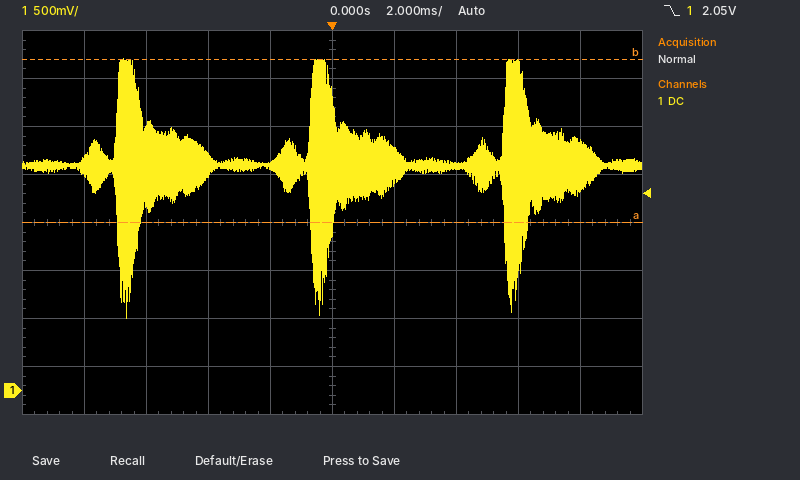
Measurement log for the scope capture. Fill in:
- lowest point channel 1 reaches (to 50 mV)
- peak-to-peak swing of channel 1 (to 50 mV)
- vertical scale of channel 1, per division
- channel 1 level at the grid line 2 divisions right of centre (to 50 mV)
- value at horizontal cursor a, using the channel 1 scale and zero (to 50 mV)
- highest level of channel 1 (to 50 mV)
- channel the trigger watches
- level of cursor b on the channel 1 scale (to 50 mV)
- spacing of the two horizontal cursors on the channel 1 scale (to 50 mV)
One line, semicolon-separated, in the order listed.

750 mV; 2.70 V; 500 mV; 2.35 V; 1.75 V; 3.45 V; channel 1; 3.45 V; 1.70 V
